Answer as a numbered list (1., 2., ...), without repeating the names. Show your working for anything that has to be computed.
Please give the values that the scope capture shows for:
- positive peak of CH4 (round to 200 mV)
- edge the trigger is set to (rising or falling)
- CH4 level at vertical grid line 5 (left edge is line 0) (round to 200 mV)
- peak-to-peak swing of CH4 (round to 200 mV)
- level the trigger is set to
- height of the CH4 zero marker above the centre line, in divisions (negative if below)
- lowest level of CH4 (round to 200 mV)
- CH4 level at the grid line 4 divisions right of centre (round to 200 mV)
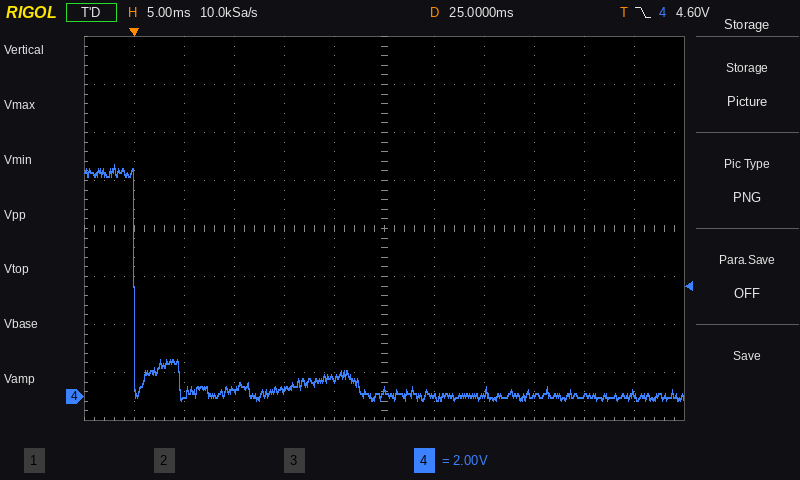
1. 9.6 V
2. falling
3. 800 mV
4. 9.6 V − (-200 mV) = 9.8 V
5. 4.60 V
6. -3.5 div
7. -200 mV
8. 0.0 V
